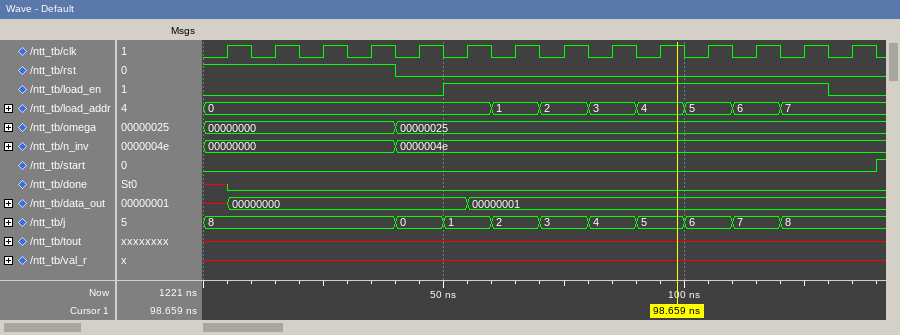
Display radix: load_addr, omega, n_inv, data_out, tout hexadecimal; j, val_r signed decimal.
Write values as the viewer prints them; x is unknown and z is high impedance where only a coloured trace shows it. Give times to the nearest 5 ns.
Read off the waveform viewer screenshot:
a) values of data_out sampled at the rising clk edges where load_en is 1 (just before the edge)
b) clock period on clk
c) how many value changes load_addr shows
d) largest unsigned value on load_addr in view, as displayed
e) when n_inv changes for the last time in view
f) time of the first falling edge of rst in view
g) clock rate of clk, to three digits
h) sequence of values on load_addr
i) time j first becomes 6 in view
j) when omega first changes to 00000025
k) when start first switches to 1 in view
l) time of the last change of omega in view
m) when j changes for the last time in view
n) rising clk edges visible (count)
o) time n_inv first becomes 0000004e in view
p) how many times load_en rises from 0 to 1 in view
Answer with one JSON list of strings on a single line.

["00000000, 00000001, 00000001, 00000001, 00000001, 00000001, 00000001, 00000001", "10 ns", "7", "7", "40 ns", "40 ns", "100 MHz", "0, 1, 2, 3, 4, 5, 6, 7", "100 ns", "40 ns", "140 ns", "40 ns", "120 ns", "14", "40 ns", "1"]
